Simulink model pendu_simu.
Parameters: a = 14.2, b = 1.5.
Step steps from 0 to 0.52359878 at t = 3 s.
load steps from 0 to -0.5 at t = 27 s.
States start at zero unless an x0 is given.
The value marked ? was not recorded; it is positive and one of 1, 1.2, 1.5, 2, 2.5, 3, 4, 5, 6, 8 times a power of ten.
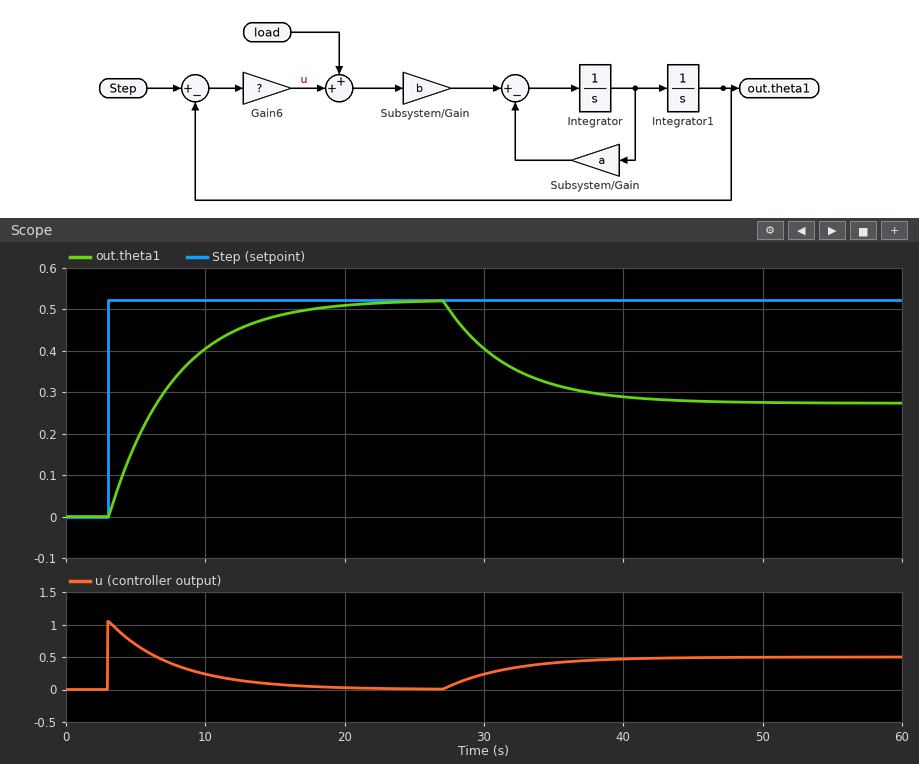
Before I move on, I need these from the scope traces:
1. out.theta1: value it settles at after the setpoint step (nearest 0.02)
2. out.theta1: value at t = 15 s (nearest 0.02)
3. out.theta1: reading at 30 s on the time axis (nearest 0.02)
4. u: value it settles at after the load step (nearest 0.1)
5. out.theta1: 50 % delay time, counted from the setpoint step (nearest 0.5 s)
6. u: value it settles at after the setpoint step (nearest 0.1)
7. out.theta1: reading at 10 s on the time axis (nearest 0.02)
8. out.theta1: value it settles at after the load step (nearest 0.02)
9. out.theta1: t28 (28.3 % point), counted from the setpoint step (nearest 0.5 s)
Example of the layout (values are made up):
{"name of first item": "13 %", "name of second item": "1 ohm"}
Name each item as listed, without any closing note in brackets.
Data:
{"out.theta1: value it settles at after the setpoint step": "0.52", "out.theta1: value at t = 15 s": "0.48", "out.theta1: reading at 30 s on the time axis": "0.40", "u: value it settles at after the load step": "0.5", "out.theta1: 50 % delay time, counted from the setpoint step": "3.5 s", "u: value it settles at after the setpoint step": "0.0", "out.theta1: reading at 10 s on the time axis": "0.40", "out.theta1: value it settles at after the load step": "0.28", "out.theta1: t28 (28.3 % point), counted from the setpoint step": "1.5 s"}
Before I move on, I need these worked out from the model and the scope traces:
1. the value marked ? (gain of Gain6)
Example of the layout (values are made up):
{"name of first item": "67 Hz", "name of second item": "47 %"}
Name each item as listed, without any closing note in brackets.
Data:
{"the value marked ?": "2"}
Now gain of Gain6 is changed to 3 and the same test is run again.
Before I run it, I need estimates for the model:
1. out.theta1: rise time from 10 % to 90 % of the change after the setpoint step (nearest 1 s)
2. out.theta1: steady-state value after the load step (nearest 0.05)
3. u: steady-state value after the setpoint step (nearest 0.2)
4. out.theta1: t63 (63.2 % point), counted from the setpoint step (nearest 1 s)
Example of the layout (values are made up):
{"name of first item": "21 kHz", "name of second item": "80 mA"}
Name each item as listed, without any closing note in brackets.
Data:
{"out.theta1: rise time from 10 % to 90 % of the change after the setpoint step": "7 s", "out.theta1: steady-state value after the load step": "0.35", "u: steady-state value after the setpoint step": "0.0", "out.theta1: t63 (63.2 % point), counted from the setpoint step": "3 s"}
